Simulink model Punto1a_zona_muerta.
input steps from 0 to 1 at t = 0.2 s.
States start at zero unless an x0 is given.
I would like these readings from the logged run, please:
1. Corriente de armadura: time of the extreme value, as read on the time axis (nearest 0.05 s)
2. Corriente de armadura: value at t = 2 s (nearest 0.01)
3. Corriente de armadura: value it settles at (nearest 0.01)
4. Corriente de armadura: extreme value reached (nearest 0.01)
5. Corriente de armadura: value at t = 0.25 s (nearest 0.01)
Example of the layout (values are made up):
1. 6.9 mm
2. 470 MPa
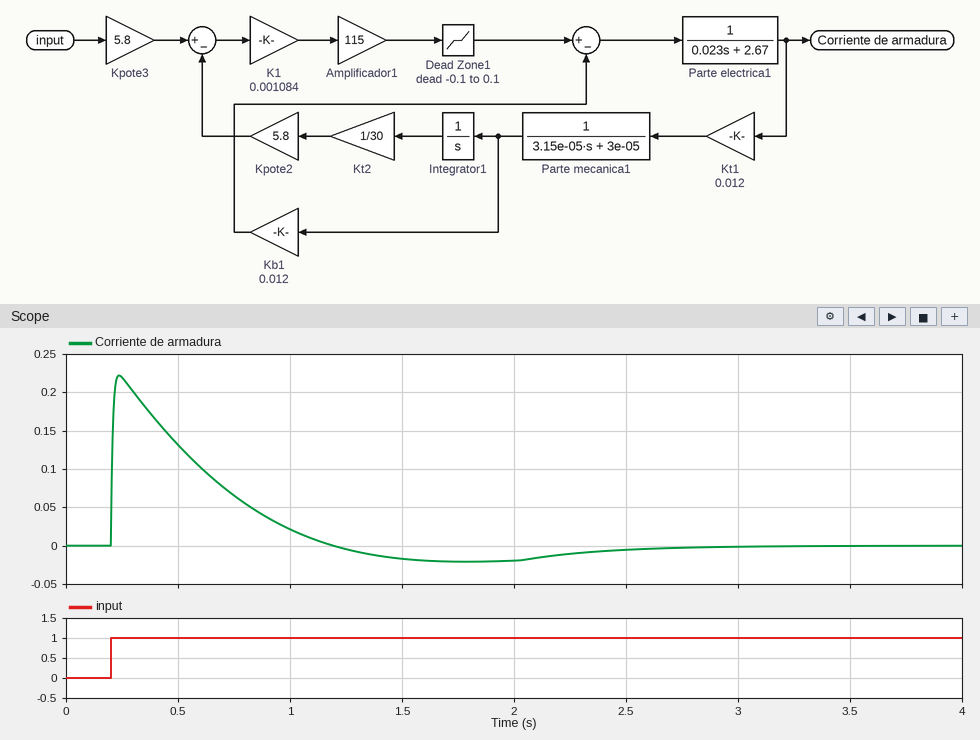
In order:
1. 0.25 s
2. -0.02
3. 0.00
4. 0.22
5. 0.22
